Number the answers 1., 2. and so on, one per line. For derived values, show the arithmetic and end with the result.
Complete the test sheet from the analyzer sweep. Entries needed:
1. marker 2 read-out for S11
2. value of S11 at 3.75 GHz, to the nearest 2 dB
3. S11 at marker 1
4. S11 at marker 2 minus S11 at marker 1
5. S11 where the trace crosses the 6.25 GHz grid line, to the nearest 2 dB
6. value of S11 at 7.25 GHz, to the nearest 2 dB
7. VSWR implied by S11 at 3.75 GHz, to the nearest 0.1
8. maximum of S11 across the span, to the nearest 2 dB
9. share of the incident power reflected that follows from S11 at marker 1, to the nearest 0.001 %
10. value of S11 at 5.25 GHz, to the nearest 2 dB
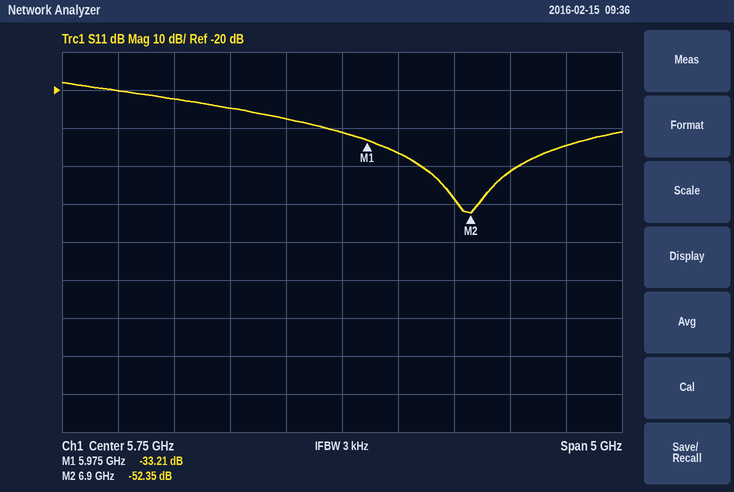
1. -52.35 dB
2. -20 dB
3. -33.21 dB
4. -52.35 − (-33.21) = -19.14 dB
5. -36 dB
6. -42 dB
7. |Γ| = 10^(-20/20) = 0.1000; VSWR = (1 + 0.1000)/(1 − 0.1000) ≈ 1.2
8. -18 dB
9. 10^(-33.21/10) ≈ 0.048 %
10. -28 dB
